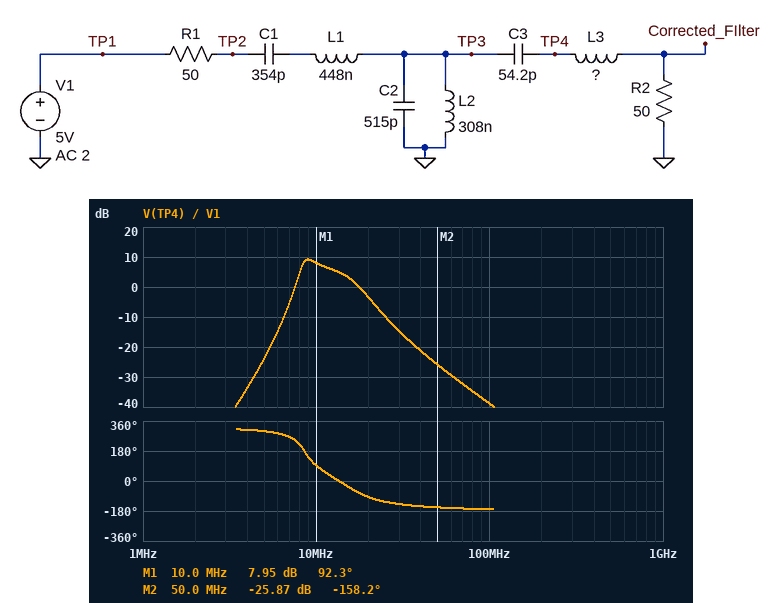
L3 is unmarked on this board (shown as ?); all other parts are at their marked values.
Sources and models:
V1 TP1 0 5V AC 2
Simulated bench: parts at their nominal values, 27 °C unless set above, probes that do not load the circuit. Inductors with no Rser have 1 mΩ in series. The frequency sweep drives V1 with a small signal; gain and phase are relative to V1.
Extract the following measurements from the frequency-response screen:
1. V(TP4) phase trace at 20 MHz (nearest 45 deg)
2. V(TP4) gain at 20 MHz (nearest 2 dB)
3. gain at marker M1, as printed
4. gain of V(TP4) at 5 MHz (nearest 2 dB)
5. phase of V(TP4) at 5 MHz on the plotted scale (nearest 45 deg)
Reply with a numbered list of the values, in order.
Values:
1. -90 deg
2. -4 dB
3. 7.95 dB
4. -24 dB
5. 315 deg
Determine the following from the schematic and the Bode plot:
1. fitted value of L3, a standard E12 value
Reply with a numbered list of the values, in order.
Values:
1. 5.6 µH
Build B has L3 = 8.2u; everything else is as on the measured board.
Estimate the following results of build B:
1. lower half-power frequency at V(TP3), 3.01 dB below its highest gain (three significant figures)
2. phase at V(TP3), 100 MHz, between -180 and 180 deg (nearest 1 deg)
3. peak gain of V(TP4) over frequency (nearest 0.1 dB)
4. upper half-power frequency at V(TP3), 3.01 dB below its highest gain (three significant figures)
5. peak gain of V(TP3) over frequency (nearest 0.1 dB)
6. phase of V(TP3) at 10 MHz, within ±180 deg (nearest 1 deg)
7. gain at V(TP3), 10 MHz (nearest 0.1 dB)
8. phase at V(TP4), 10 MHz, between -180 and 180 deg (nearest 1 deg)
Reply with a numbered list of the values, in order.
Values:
1. 9.80 MHz
2. -170 deg
3. 8.5 dB
4. 17.9 MHz
5. -0.1 dB
6. 61 deg
7. -2.7 dB
8. 69 deg
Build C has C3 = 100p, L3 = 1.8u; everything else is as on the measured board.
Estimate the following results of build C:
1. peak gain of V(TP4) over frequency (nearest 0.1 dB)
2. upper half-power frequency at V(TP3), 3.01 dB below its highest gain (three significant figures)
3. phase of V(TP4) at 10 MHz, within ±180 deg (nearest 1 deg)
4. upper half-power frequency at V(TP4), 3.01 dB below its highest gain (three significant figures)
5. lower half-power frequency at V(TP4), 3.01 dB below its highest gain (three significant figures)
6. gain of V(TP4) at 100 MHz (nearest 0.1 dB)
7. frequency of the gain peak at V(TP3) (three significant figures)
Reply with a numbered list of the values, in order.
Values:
1. 4.1 dB
2. 20.2 MHz
3. 134 deg
4. 18.6 MHz
5. 9.74 MHz
6. -38.8 dB
7. 16.6 MHz
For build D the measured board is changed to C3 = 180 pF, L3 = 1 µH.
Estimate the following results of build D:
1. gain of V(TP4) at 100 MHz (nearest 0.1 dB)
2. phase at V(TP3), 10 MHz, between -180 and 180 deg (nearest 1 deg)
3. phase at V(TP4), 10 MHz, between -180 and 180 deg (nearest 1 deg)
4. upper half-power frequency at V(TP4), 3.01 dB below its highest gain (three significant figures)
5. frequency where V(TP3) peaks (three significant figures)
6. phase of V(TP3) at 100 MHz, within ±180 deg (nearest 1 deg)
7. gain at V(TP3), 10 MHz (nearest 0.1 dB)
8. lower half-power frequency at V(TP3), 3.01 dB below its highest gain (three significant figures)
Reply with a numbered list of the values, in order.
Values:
1. -38.8 dB
2. 27 deg
3. 106 deg
4. 20.5 MHz
5. 17.5 MHz
6. -170 deg
7. -5.1 dB
8. 7.43 MHz
